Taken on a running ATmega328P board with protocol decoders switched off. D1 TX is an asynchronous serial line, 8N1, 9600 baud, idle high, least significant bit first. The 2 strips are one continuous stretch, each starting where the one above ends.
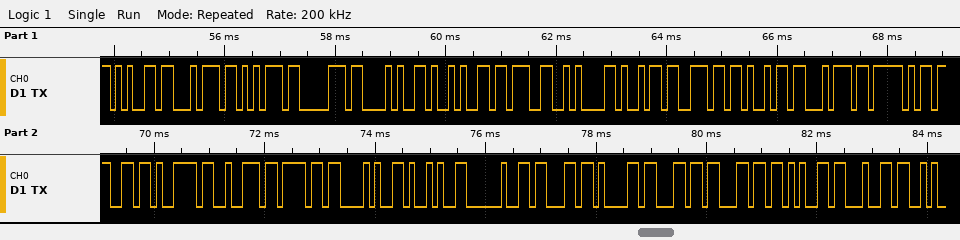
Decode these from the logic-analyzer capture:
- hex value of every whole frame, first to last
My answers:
0x65 0x74 0x75 0x70 0x28 0x29 0x3B 0x0A 0x69 0x6E 0x69 0x74 0x5F 0x67 0x79 0x72 0x6F 0x28 0x29 0x20 0x63 0x61 0x6C 0x6C 0x65 0x64
